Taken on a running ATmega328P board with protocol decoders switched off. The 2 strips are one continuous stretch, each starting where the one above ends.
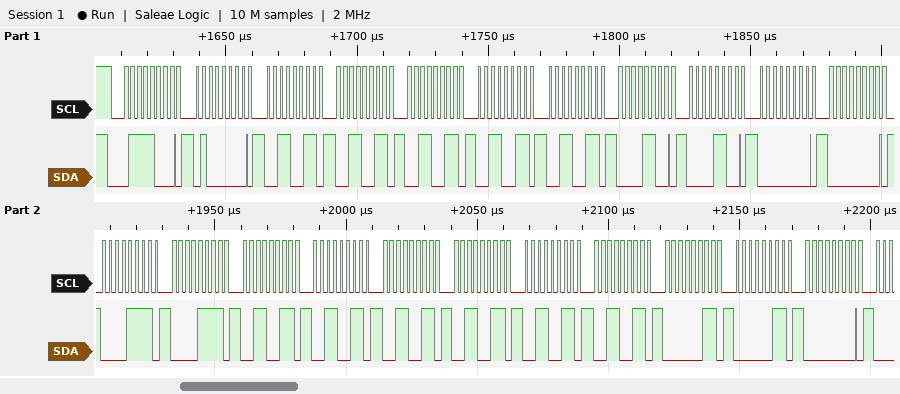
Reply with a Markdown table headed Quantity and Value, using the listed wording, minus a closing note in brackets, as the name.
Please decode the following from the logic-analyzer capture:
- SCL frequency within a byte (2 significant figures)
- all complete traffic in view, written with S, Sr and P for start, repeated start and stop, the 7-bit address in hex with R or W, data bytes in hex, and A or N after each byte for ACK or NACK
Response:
| Quantity | Value |
|---|---|
| SCL frequency within a byte | 400 kHz |
| all complete traffic in view, written with S, Sr and P for start, repeated start and stop, the 7-bit address in hex with R or W, data bytes in hex, and A or N after each byte for ACK or NACK | S 3CW A 40 A 33 A 33 A 33 A 33 A 33 A 0C A 0C A 00 A 00 A 0F A 0F A 33 A 33 A 33 A 33 A 33 A 33 A 03 A 03 A 00 A |
